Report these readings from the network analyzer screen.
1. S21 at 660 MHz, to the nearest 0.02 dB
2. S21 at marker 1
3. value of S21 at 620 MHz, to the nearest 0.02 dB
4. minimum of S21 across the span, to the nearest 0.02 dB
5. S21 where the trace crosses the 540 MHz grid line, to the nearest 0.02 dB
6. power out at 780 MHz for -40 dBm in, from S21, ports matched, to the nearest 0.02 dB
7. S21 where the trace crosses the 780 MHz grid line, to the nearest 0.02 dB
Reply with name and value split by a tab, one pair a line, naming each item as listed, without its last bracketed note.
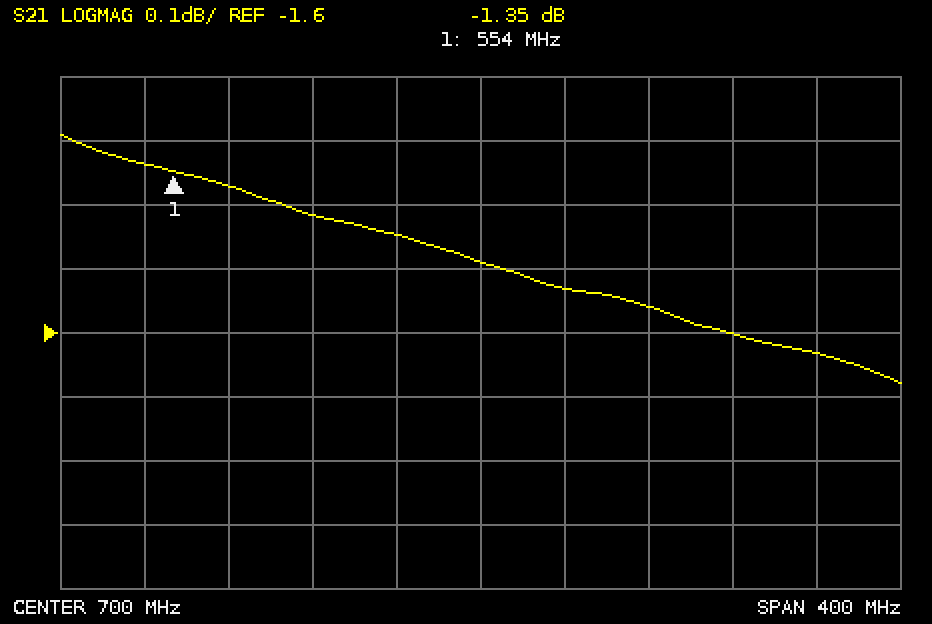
S21 at 660 MHz, to the nearest 0.02 dB	-1.44 dB
S21 at marker 1	-1.35 dB
value of S21 at 620 MHz, to the nearest 0.02 dB	-1.42 dB
minimum of S21 across the span, to the nearest 0.02 dB	-1.68 dB
S21 where the trace crosses the 540 MHz grid line, to the nearest 0.02 dB	-1.34 dB
power out at 780 MHz for -40 dBm in, from S21, ports matched, to the nearest 0.02 dB	-41.56 dBm
S21 where the trace crosses the 780 MHz grid line, to the nearest 0.02 dB	-1.56 dB
